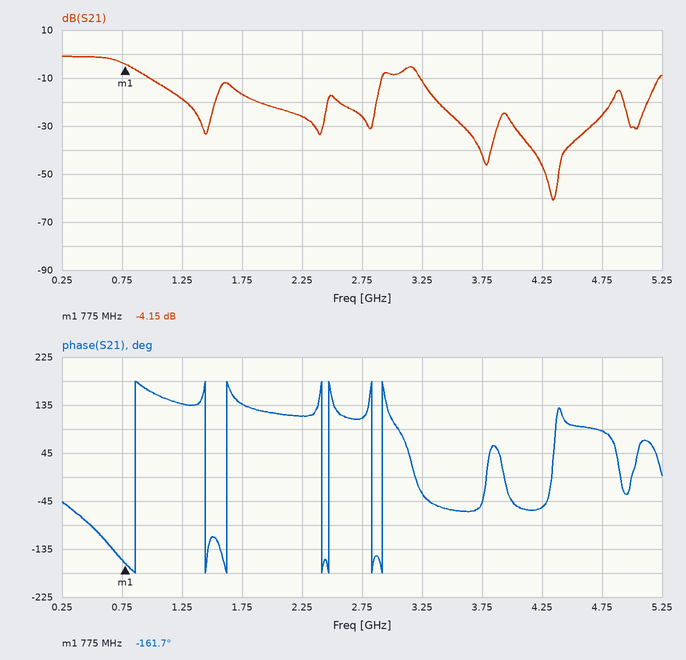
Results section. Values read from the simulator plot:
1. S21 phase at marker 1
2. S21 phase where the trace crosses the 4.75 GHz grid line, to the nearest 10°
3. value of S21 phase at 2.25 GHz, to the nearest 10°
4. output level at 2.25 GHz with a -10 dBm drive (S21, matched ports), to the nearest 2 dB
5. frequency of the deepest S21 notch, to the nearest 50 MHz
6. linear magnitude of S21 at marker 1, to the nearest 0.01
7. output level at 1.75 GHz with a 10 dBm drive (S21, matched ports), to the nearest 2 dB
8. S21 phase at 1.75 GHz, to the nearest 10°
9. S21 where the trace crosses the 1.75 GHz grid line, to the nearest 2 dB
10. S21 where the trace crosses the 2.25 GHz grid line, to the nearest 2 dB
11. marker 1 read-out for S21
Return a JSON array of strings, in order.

["-161.7°", "90°", "110°", "-36 dBm", "4.35 GHz", "0.62", "-6 dBm", "140°", "-16 dB", "-26 dB", "-4.15 dB"]
